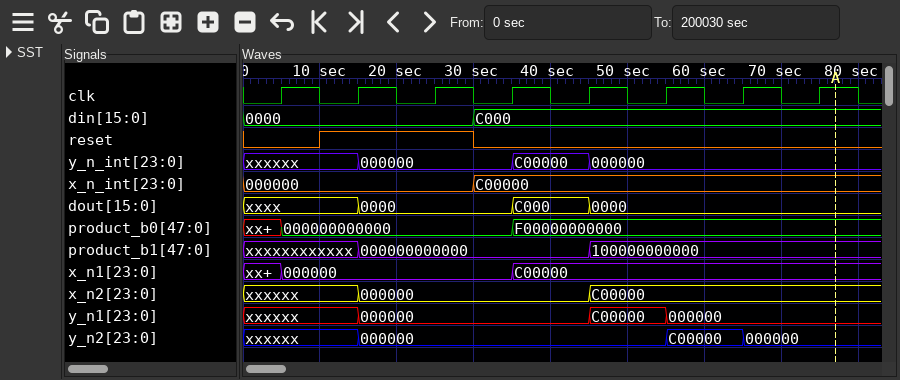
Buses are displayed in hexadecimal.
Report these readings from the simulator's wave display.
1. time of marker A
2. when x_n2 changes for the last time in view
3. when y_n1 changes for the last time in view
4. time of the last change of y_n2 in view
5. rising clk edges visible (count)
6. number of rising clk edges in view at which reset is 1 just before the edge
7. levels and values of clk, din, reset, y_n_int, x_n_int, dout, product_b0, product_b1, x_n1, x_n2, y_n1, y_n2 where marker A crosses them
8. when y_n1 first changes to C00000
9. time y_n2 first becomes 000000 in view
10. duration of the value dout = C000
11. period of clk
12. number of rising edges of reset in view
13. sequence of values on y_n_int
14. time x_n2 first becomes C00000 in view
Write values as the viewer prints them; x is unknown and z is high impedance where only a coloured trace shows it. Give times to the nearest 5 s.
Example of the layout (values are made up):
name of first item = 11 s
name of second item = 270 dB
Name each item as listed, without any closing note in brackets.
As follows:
time of marker A = 75 s
when x_n2 changes for the last time in view = 45 s
when y_n1 changes for the last time in view = 55 s
time of the last change of y_n2 in view = 65 s
rising clk edges visible = 8
number of rising clk edges in view at which reset is 1 just before the edge = 2
levels and values of clk, din, reset, y_n_int, x_n_int, dout, product_b0, product_b1, x_n1, x_n2, y_n1, y_n2 where marker A crosses them = clk=1, din=C000, reset=0, y_n_int=000000, x_n_int=C00000, dout=0000, product_b0=F00000000000, product_b1=100000000000, x_n1=C00000, x_n2=C00000, y_n1=000000, y_n2=000000
when y_n1 first changes to C00000 = 45 s
time y_n2 first becomes 000000 in view = 15 s
duration of the value dout = C000 = 10 s
period of clk = 10 s
number of rising edges of reset in view = 1
sequence of values on y_n_int = xxxxxx, 000000, C00000, 000000
time x_n2 first becomes C00000 in view = 45 s
